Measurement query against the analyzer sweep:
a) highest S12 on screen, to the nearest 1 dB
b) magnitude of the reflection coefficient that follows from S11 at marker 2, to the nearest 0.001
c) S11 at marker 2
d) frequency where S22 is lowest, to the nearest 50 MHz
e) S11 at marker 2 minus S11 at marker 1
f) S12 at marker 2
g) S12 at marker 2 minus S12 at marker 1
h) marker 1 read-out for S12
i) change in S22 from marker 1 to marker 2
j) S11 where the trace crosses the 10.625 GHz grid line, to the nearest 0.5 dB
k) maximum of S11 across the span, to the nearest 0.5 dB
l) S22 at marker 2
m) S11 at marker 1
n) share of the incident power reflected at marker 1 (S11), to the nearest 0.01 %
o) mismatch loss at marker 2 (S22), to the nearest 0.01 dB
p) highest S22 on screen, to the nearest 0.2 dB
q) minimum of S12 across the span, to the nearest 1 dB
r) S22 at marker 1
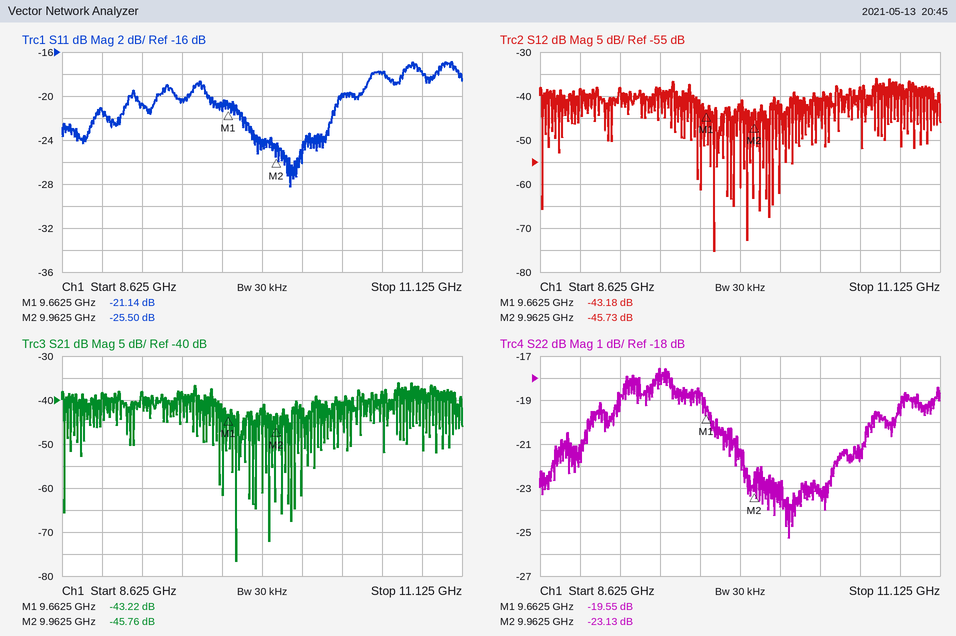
-36 dB
0.053
-25.50 dB
10.20 GHz
-4.36 dB
-45.73 dB
-2.55 dB
-43.18 dB
-3.58 dB
-18.0 dB
-17.0 dB
-23.13 dB
-21.14 dB
0.77 %
0.02 dB
-17.6 dB
-75 dB
-19.55 dB
